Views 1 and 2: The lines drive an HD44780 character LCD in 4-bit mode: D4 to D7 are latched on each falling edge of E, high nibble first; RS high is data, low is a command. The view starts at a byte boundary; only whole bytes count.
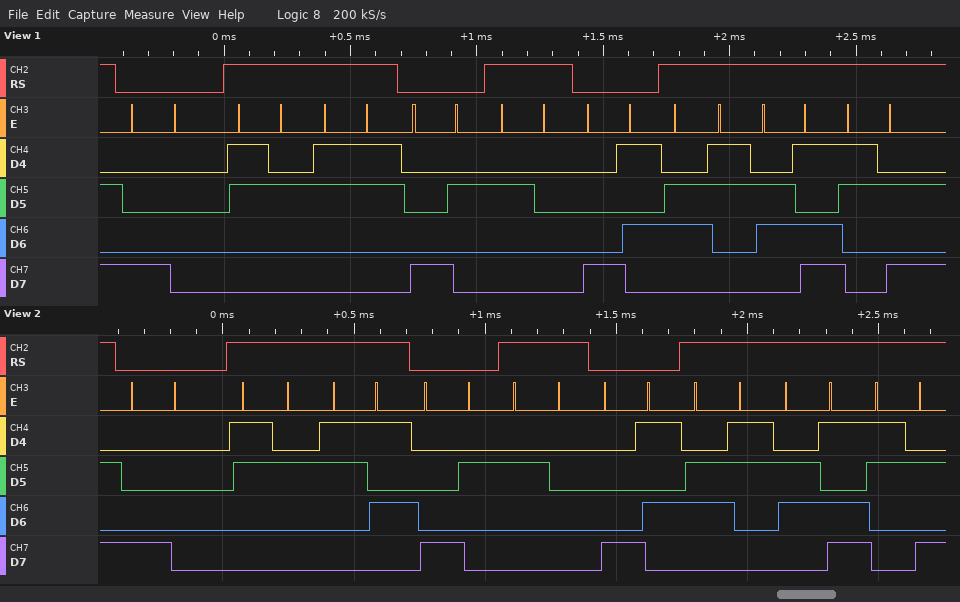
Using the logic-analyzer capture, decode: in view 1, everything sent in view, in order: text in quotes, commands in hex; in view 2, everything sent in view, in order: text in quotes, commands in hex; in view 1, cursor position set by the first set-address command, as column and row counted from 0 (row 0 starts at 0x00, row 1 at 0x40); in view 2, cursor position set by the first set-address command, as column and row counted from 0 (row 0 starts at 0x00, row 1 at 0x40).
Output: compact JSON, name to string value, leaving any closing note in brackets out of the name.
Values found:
{"in view 1, everything sent in view, in order: text in quotes, commands in hex": "0x80 \"23\" 0x82 \" \" 0x85 \"cm:\"", "in view 2, everything sent in view, in order: text in quotes, commands in hex": "0x80 \"25\" 0x82 \" \" 0x85 \"cm:\"", "in view 1, cursor position set by the first set-address command, as column and row counted from 0": "column 0, row 0", "in view 2, cursor position set by the first set-address command, as column and row counted from 0": "column 0, row 0"}
